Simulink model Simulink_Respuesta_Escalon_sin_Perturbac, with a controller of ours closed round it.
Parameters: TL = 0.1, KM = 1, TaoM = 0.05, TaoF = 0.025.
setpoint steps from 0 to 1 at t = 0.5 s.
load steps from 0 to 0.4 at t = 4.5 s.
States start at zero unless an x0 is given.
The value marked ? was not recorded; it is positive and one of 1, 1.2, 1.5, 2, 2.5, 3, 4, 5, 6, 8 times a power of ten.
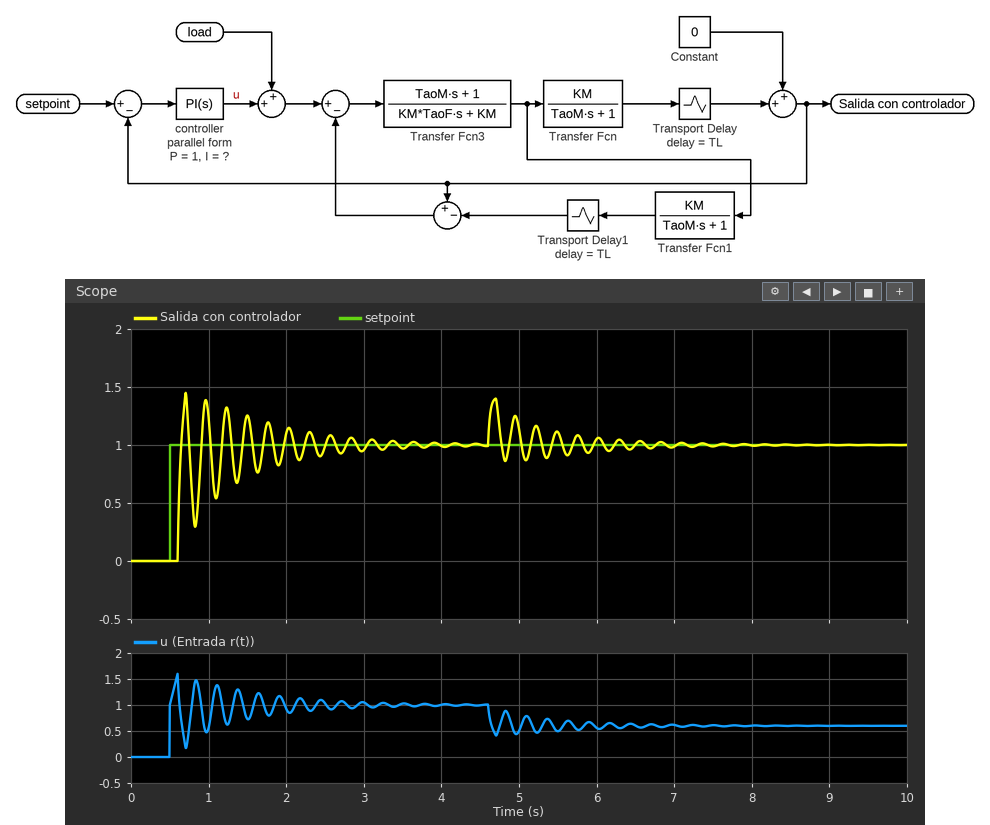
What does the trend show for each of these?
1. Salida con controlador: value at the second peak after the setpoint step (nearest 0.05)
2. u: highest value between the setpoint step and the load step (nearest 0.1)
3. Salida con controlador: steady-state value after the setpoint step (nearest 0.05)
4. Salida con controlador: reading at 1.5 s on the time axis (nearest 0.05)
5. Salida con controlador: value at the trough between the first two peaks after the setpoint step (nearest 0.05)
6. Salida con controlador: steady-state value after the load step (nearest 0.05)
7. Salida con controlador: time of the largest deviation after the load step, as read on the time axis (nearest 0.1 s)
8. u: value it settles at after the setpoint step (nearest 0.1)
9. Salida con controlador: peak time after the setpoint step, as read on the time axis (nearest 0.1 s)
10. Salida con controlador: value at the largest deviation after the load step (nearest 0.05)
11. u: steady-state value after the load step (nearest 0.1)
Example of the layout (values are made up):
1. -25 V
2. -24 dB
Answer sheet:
1. 1.40
2. 1.6
3. 1.00
4. 1.25
5. 0.30
6. 1.00
7. 4.7 s
8. 1.0
9. 0.7 s
10. 1.40
11. 0.6
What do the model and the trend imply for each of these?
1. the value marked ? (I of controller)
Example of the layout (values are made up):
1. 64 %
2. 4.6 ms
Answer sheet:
1. 6
